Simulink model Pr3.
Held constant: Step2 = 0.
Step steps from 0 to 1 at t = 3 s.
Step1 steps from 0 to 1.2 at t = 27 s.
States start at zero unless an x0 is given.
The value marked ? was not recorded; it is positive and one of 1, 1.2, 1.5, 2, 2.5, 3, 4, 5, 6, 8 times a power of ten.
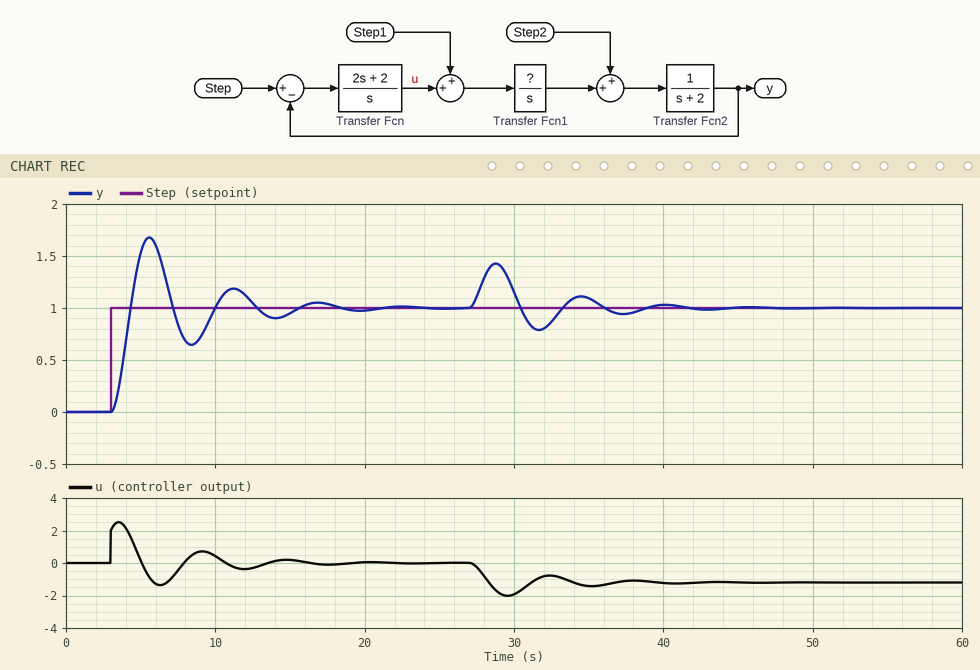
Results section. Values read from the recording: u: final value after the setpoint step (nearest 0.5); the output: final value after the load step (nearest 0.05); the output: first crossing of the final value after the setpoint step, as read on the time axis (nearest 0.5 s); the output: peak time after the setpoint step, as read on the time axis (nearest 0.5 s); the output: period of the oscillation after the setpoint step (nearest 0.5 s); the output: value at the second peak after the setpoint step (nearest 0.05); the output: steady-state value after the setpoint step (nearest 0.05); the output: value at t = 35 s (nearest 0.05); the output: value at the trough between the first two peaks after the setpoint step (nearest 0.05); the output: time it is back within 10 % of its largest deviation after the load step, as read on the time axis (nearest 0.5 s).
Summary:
0.0
1.00
4.5 s
5.5 s
5.5 s
1.20
1.00
1.10
0.65
38.0 s
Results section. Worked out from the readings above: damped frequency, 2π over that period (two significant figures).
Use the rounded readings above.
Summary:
1.1 rad/s
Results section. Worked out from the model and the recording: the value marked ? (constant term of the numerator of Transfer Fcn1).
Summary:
1
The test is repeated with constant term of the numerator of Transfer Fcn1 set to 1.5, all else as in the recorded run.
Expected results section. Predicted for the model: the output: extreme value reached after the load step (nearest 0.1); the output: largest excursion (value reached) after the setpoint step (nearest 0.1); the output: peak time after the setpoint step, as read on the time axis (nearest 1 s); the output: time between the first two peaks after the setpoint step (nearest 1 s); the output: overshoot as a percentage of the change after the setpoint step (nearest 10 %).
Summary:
1.5
1.7
5 s
4 s
70 %
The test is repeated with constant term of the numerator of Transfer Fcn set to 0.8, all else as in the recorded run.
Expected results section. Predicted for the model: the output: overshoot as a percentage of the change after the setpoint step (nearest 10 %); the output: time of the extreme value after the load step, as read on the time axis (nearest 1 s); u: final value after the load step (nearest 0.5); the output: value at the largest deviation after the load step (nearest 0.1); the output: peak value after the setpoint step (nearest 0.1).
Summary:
40 %
29 s
-1.0
1.5
1.4
